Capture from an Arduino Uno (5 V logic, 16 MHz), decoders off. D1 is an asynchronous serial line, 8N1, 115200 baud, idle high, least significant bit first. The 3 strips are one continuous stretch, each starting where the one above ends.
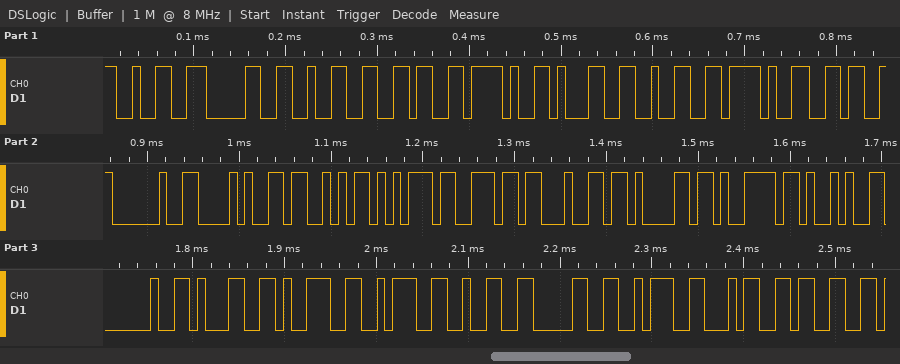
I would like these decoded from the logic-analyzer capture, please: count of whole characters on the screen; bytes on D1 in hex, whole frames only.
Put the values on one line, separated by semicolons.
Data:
27; 32 30 32 36 2F 31 32 2F 36 20 28 53 75 6E 64 61 79 29 20 31 39 3A 32 30 3A 34 33
